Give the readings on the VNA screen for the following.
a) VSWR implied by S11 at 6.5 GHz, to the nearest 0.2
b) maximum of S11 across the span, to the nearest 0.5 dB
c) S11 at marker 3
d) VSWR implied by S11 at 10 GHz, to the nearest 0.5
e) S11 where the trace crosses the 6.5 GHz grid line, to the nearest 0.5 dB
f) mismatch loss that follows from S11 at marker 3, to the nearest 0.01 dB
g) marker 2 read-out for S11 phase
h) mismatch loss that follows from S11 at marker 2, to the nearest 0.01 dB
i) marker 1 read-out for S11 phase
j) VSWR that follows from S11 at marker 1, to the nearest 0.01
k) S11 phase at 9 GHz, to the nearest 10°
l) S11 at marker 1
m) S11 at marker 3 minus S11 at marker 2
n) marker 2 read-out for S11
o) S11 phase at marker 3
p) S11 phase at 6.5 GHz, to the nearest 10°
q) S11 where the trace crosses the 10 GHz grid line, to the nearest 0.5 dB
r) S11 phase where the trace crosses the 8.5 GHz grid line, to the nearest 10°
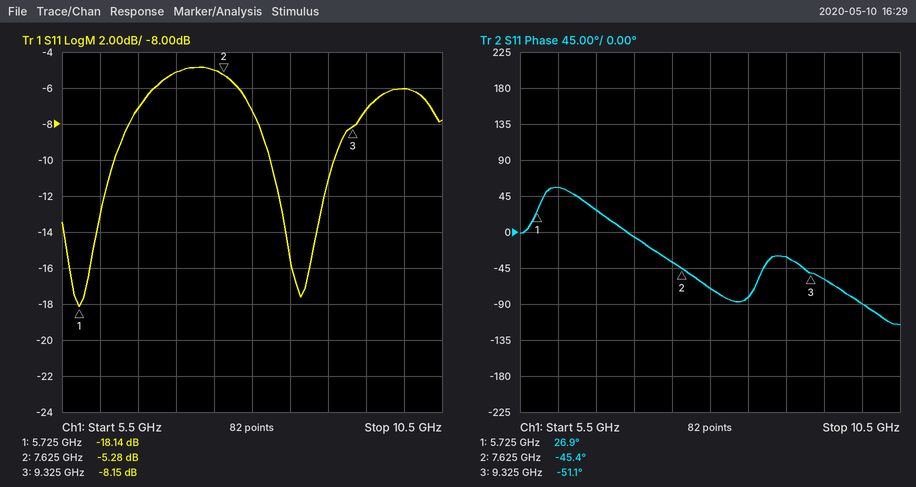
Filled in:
2.6
-5.0 dB
-8.15 dB
3.0
-7.0 dB
0.72 dB
-45.4°
1.53 dB
26.9°
1.28
-30°
-18.14 dB
-2.87 dB
-5.28 dB
-51.1°
30°
-6.0 dB
-80°
